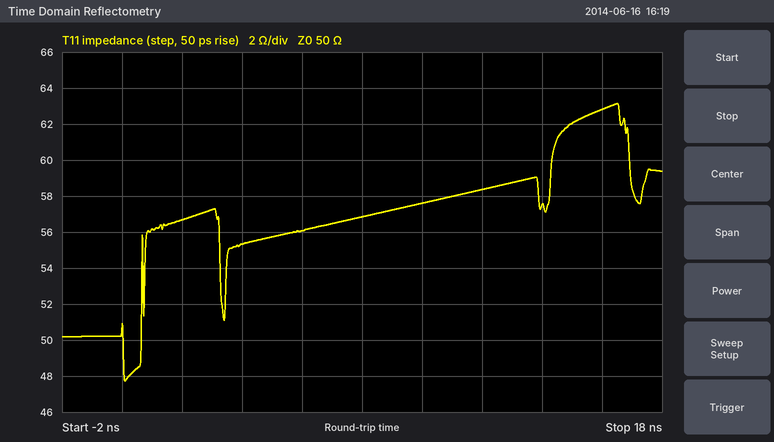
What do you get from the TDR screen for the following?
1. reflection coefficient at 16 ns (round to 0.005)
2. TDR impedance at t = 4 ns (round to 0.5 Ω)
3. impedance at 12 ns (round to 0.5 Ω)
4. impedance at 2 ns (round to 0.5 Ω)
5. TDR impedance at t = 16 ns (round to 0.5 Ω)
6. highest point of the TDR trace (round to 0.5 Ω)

+0.115
55.5 Ω
58.5 Ω
56.5 Ω
63.0 Ω
63.0 Ω
